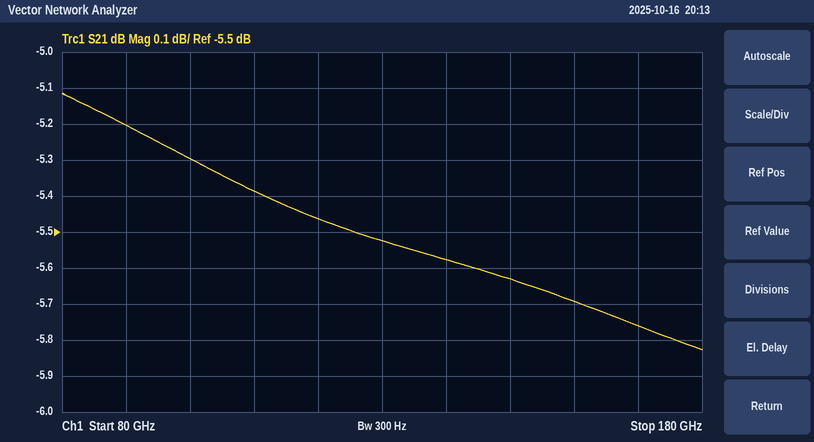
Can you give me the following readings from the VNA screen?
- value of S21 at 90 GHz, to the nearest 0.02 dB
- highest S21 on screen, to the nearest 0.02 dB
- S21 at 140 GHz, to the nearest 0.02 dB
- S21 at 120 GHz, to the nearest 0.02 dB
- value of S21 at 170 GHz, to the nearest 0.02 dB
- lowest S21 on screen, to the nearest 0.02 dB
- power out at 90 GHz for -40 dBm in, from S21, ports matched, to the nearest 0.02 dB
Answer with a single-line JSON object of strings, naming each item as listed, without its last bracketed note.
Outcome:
{"value of S21 at 90 GHz, to the nearest 0.02 dB": "-5.20 dB", "highest S21 on screen, to the nearest 0.02 dB": "-5.12 dB", "S21 at 140 GHz, to the nearest 0.02 dB": "-5.58 dB", "S21 at 120 GHz, to the nearest 0.02 dB": "-5.46 dB", "value of S21 at 170 GHz, to the nearest 0.02 dB": "-5.76 dB", "lowest S21 on screen, to the nearest 0.02 dB": "-5.82 dB", "power out at 90 GHz for -40 dBm in, from S21, ports matched, to the nearest 0.02 dB": "-45.20 dBm"}
